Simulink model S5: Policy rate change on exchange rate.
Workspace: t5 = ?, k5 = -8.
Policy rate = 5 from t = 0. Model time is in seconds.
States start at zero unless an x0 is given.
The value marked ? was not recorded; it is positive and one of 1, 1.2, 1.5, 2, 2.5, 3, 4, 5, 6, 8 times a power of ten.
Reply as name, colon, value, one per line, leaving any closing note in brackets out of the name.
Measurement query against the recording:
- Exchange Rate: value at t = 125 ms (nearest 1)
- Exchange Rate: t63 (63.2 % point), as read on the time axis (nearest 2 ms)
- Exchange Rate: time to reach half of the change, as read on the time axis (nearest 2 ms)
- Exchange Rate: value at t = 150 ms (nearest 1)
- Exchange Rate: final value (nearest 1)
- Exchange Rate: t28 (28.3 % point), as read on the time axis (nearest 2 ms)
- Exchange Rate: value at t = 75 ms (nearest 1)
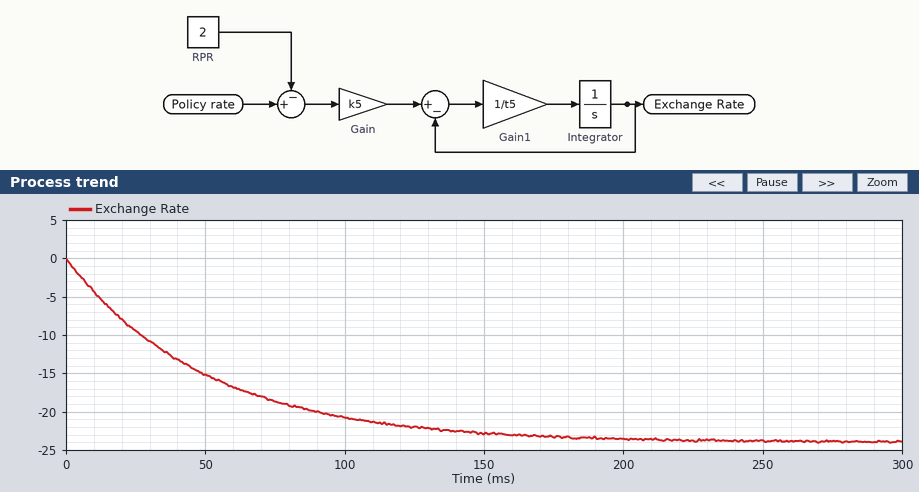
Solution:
Exchange Rate: value at t = 125 ms: -22
Exchange Rate: t63 (63.2 % point), as read on the time axis: 50 ms
Exchange Rate: time to reach half of the change, as read on the time axis: 34 ms
Exchange Rate: value at t = 150 ms: -23
Exchange Rate: final value: -24
Exchange Rate: t28 (28.3 % point), as read on the time axis: 16 ms
Exchange Rate: value at t = 75 ms: -19
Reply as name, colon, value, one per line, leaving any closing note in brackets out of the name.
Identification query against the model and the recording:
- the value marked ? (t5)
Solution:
the value marked ?: 0.05
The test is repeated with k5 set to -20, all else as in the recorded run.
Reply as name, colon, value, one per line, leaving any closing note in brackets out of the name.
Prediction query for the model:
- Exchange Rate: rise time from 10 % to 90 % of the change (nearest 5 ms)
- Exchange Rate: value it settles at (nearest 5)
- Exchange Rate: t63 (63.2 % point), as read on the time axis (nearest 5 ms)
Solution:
Exchange Rate: rise time from 10 % to 90 % of the change: 110 ms
Exchange Rate: value it settles at: -60
Exchange Rate: t63 (63.2 % point), as read on the time axis: 50 ms
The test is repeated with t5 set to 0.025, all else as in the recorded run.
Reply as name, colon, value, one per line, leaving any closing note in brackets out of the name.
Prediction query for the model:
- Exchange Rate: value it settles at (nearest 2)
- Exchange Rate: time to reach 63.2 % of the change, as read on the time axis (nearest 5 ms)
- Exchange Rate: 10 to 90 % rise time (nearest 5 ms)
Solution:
Exchange Rate: value it settles at: -24
Exchange Rate: time to reach 63.2 % of the change, as read on the time axis: 25 ms
Exchange Rate: 10 to 90 % rise time: 55 ms
